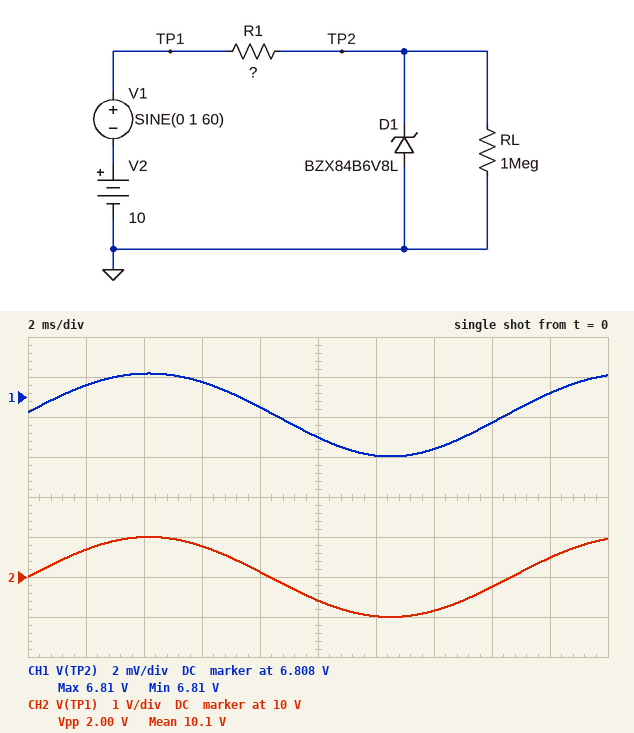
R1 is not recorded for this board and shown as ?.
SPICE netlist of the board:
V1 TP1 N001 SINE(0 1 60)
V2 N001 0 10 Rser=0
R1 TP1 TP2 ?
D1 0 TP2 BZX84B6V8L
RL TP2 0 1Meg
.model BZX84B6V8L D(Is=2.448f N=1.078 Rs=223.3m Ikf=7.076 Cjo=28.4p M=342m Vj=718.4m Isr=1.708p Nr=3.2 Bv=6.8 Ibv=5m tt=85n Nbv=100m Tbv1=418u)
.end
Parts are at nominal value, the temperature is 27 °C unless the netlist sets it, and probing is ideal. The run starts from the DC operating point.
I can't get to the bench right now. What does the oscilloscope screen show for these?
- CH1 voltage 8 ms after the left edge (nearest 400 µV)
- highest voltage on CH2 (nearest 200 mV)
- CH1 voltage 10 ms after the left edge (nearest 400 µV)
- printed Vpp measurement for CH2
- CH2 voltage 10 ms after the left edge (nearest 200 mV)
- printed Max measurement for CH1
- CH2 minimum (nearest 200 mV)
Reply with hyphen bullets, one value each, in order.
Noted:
- 6.8076 V
- 11.0 V
- 6.8060 V
- 2.00 V
- 9.4 V
- 6.81 V
- 9.0 V
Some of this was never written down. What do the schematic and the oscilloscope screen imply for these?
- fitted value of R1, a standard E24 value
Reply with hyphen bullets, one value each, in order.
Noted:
- 180 Ω
